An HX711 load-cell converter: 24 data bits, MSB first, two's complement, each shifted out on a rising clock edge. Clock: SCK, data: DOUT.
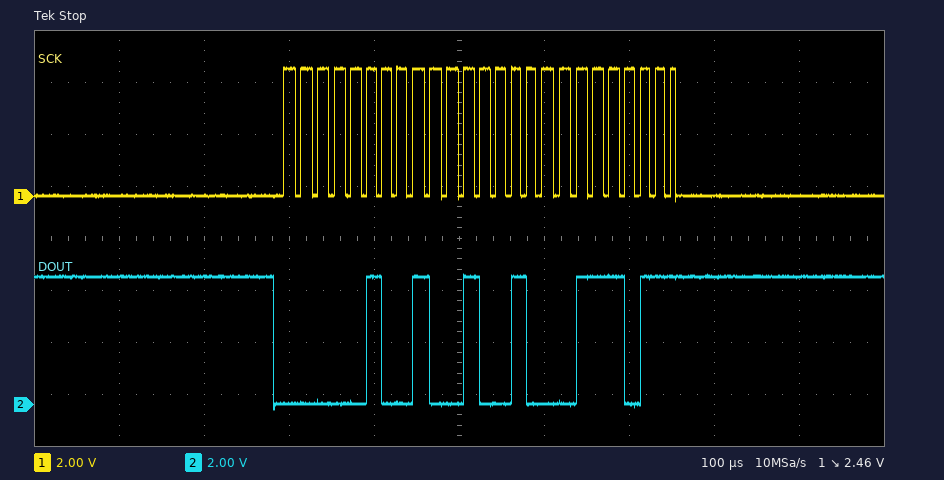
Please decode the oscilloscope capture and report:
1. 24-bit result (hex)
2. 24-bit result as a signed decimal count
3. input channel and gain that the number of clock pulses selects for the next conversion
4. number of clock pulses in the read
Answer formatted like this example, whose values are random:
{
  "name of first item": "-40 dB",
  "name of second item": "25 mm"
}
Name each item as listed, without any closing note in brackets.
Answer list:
{
  "24-bit result": "0x04923B",
  "24-bit result as a signed decimal count": "299579",
  "input channel and gain that the number of clock pulses selects for the next conversion": "channel A, gain 128",
  "number of clock pulses in the read": "25"
}
